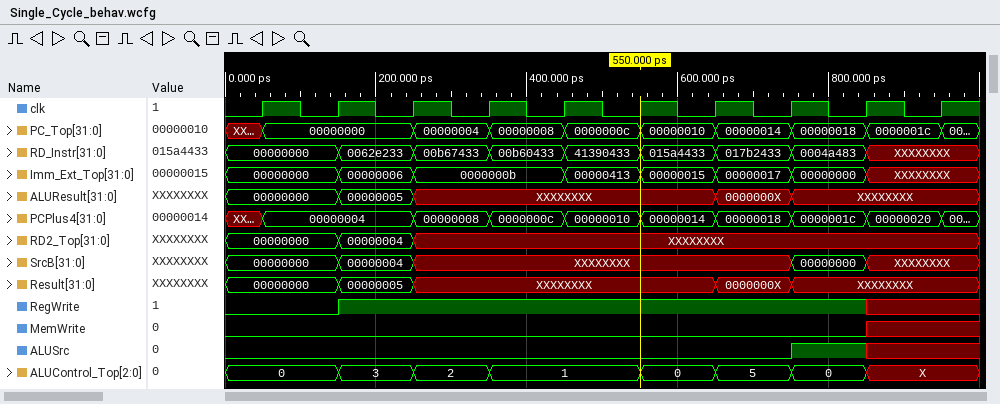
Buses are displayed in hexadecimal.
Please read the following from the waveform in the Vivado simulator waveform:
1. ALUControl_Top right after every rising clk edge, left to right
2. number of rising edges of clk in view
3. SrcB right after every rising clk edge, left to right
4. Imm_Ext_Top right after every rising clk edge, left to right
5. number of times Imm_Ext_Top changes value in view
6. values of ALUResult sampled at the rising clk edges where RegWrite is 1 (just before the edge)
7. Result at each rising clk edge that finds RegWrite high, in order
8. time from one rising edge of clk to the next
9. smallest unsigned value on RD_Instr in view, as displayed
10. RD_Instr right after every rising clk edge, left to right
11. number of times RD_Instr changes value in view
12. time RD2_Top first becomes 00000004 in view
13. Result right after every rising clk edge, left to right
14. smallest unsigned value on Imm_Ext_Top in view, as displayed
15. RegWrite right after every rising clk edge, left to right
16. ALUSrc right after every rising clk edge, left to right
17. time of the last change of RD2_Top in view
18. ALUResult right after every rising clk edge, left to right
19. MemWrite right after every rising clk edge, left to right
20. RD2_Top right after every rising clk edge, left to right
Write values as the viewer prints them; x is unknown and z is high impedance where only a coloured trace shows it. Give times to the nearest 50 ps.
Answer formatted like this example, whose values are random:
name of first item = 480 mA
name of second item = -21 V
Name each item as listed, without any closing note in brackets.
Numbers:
ALUControl_Top right after every rising clk edge, left to right = 0, 3, 2, 1, 1, 0, 5, 0, X, X
number of rising edges of clk in view = 10
SrcB right after every rising clk edge, left to right = 00000000, 00000004, XXXXXXXX, XXXXXXXX, XXXXXXXX, XXXXXXXX, XXXXXXXX, 00000000, XXXXXXXX, XXXXXXXX
Imm_Ext_Top right after every rising clk edge, left to right = 00000000, 00000006, 0000000b, 0000000b, 00000413, 00000015, 00000017, 00000000, XXXXXXXX, XXXXXXXX
number of times Imm_Ext_Top changes value in view = 7
values of ALUResult sampled at the rising clk edges where RegWrite is 1 = 00000005, XXXXXXXX, XXXXXXXX, XXXXXXXX, XXXXXXXX, 0000000X, XXXXXXXX
Result at each rising clk edge that finds RegWrite high, in order = 00000005, XXXXXXXX, XXXXXXXX, XXXXXXXX, XXXXXXXX, 0000000X, XXXXXXXX
time from one rising edge of clk to the next = 100 ps
smallest unsigned value on RD_Instr in view, as displayed = 00000000
RD_Instr right after every rising clk edge, left to right = 00000000, 0062e233, 00b67433, 00b60433, 41390433, 015a4433, 017b2433, 0004a483, XXXXXXXX, XXXXXXXX
number of times RD_Instr changes value in view = 8
time RD2_Top first becomes 00000004 in view = 150 ps
Result right after every rising clk edge, left to right = 00000000, 00000005, XXXXXXXX, XXXXXXXX, XXXXXXXX, XXXXXXXX, 0000000X, XXXXXXXX, XXXXXXXX, XXXXXXXX
smallest unsigned value on Imm_Ext_Top in view, as displayed = 00000000
RegWrite right after every rising clk edge, left to right = 0 1 1 1 1 1 1 1 x x
ALUSrc right after every rising clk edge, left to right = 0 0 0 0 0 0 0 1 x x
time of the last change of RD2_Top in view = 250 ps
ALUResult right after every rising clk edge, left to right = 00000000, 00000005, XXXXXXXX, XXXXXXXX, XXXXXXXX, XXXXXXXX, 0000000X, XXXXXXXX, XXXXXXXX, XXXXXXXX
MemWrite right after every rising clk edge, left to right = 0 0 0 0 0 0 0 0 x x
RD2_Top right after every rising clk edge, left to right = 00000000, 00000004, XXXXXXXX, XXXXXXXX, XXXXXXXX, XXXXXXXX, XXXXXXXX, XXXXXXXX, XXXXXXXX, XXXXXXXX
